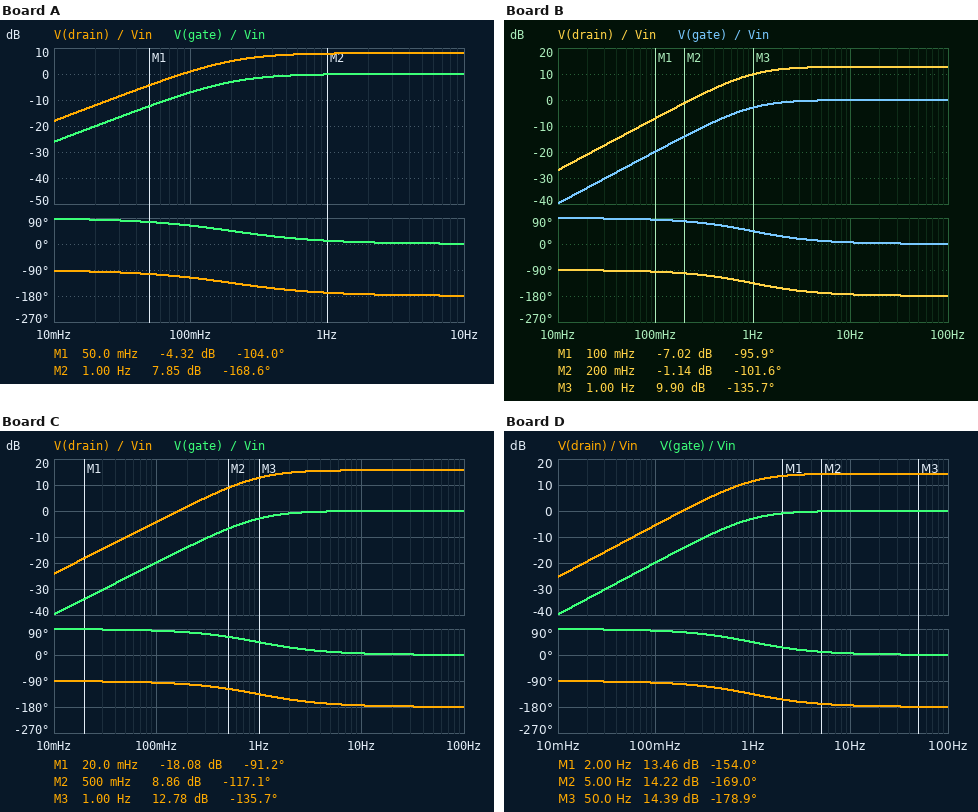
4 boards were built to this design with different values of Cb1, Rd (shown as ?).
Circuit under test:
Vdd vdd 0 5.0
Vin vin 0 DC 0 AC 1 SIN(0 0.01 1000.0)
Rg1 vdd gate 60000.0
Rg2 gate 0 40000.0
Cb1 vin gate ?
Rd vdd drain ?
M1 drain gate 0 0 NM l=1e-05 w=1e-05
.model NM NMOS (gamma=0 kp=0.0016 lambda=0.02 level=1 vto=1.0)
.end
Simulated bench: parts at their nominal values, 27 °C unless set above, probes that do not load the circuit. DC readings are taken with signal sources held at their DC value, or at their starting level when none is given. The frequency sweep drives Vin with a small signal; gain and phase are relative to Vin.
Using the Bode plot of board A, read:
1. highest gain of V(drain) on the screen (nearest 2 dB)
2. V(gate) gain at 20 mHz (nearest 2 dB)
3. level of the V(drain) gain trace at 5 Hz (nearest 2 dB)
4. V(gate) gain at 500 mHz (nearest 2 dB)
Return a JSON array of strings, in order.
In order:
["8 dB", "-20 dB", "8 dB", "0 dB"]
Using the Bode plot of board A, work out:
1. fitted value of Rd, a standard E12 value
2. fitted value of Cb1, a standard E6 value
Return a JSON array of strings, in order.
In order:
["1.5 kΩ", "33 µF"]
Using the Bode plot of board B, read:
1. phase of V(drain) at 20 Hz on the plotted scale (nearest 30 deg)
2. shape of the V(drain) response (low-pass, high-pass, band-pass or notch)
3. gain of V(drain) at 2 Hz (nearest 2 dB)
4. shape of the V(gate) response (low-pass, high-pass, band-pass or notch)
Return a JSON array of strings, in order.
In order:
["-180 deg", "high-pass", "12 dB", "high-pass"]
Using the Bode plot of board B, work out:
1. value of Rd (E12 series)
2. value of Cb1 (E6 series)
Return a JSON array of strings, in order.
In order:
["2.7 kΩ", "6.8 µF"]
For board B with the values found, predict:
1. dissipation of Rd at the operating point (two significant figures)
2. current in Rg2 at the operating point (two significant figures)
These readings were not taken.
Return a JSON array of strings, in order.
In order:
["1.9 mW", "50 µA"]
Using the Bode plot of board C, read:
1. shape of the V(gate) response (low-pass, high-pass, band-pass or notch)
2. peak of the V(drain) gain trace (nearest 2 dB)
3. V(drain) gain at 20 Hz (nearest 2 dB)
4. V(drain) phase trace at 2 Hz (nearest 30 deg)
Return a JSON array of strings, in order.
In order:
["high-pass", "16 dB", "16 dB", "-150 deg"]
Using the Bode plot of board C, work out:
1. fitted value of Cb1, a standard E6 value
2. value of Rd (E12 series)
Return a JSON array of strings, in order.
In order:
["6.8 µF", "3.9 kΩ"]
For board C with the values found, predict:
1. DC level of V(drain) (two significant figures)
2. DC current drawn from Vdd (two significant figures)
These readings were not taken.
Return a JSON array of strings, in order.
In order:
["1.8 V", "880 µA"]
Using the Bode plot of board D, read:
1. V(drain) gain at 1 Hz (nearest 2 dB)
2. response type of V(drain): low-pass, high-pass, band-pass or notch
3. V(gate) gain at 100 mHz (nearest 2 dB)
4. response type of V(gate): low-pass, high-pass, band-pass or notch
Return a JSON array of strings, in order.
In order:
["12 dB", "high-pass", "-20 dB", "high-pass"]
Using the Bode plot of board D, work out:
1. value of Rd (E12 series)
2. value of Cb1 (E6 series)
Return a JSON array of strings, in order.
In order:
["3.3 kΩ", "6.8 µF"]
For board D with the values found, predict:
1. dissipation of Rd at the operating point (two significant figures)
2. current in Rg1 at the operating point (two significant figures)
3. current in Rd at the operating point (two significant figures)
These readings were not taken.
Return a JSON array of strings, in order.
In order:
["2.3 mW", "50 µA", "840 µA"]
